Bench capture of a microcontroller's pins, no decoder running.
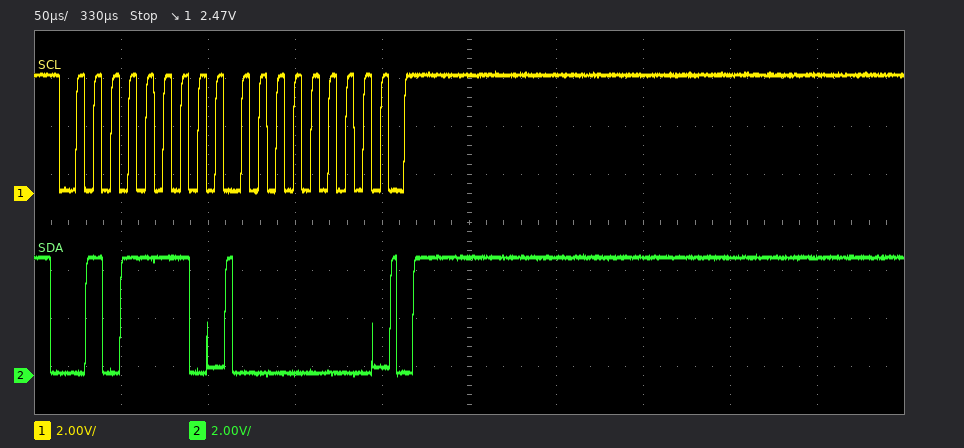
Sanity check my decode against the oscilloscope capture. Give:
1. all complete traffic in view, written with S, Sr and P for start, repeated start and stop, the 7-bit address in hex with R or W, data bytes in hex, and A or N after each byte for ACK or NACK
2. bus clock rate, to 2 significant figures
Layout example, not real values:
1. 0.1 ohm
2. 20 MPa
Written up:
1. S 2FW A 00 A P
2. 100 kHz
